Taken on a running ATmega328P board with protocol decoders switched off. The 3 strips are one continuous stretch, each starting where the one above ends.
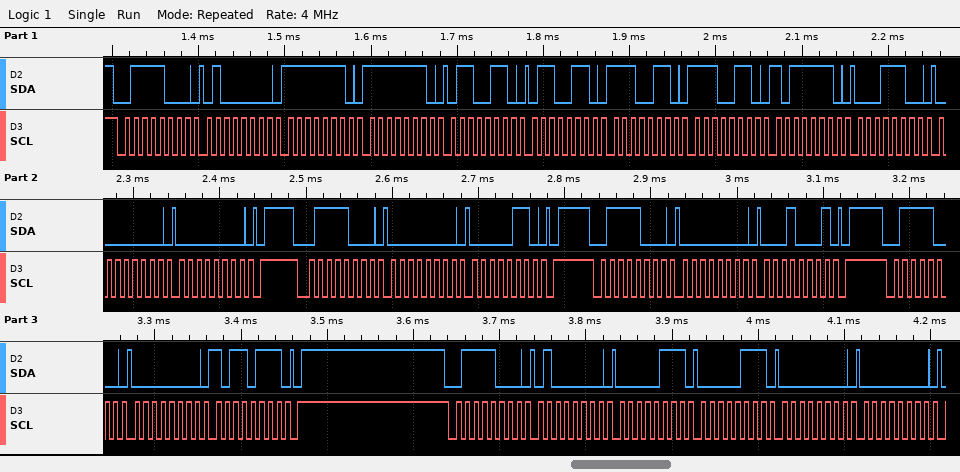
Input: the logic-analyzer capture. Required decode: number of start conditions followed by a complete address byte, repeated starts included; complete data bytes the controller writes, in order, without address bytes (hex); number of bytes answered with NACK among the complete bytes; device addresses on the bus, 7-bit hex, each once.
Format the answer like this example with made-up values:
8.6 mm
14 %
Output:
5
40 FE FE 66 66 E6 E6 BE 1C 00 00 00 06 00 11 00 B7 40 07 07 00 00
0
0x3C
